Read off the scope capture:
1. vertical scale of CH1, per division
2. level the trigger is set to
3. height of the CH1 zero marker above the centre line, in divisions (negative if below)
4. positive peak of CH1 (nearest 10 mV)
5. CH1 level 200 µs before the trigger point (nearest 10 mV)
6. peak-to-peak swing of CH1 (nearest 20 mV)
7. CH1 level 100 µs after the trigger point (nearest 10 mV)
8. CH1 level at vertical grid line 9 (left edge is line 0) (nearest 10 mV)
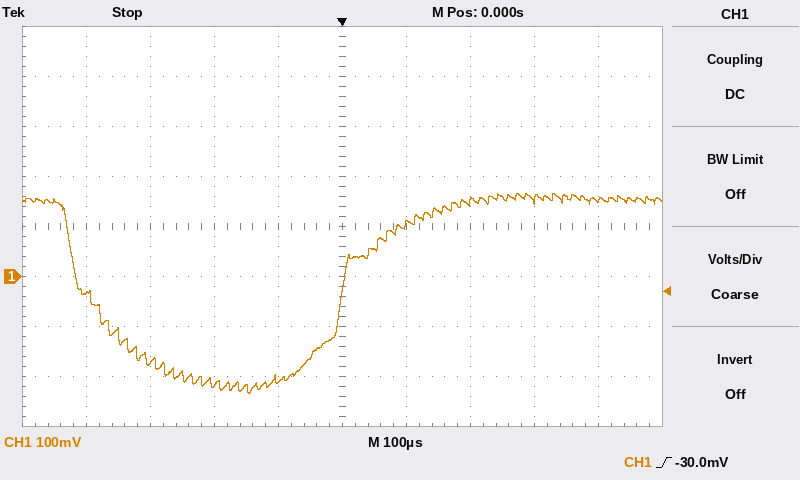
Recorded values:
100 mV
-30.0 mV
-1.0 div
170 mV
-220 mV
400 mV
100 mV
150 mV
